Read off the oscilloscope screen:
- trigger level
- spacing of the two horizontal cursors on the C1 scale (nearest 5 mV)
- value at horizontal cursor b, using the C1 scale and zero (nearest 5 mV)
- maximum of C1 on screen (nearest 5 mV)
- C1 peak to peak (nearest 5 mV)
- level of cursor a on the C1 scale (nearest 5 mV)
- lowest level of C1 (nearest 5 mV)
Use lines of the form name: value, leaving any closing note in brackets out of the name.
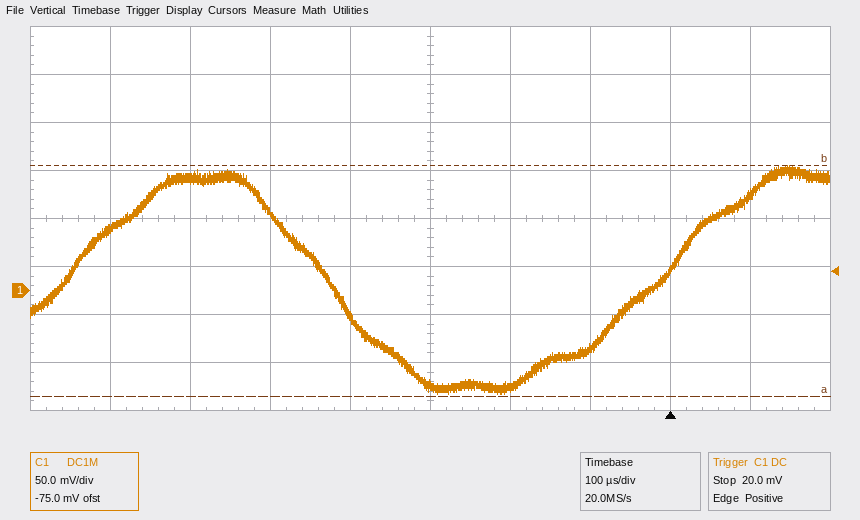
trigger level: 20.0 mV
spacing of the two horizontal cursors on the C1 scale: 240 mV
value at horizontal cursor b, using the C1 scale and zero: 130 mV
maximum of C1 on screen: 130 mV
C1 peak to peak: 240 mV
level of cursor a on the C1 scale: -110 mV
lowest level of C1: -110 mV
